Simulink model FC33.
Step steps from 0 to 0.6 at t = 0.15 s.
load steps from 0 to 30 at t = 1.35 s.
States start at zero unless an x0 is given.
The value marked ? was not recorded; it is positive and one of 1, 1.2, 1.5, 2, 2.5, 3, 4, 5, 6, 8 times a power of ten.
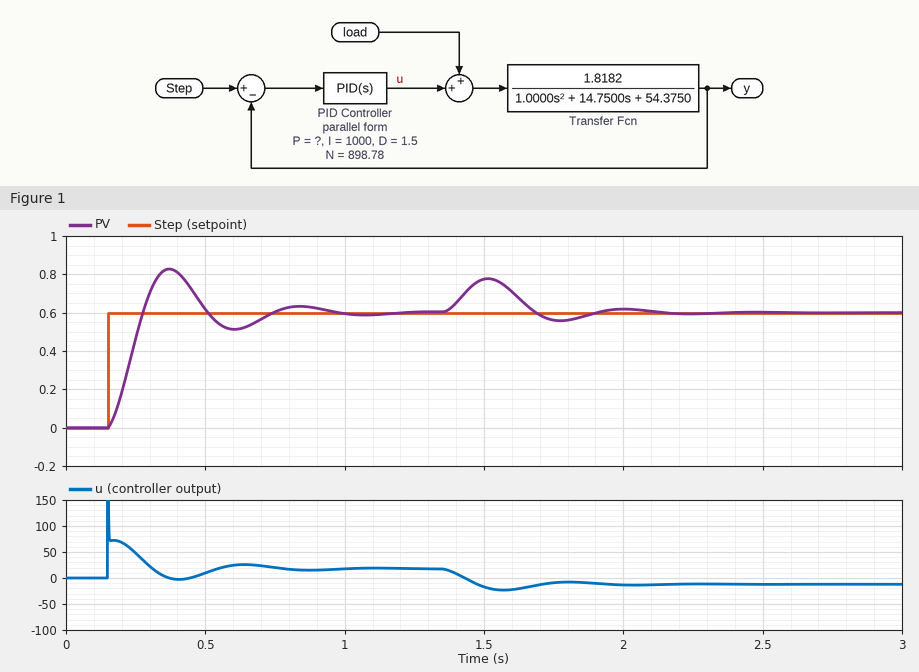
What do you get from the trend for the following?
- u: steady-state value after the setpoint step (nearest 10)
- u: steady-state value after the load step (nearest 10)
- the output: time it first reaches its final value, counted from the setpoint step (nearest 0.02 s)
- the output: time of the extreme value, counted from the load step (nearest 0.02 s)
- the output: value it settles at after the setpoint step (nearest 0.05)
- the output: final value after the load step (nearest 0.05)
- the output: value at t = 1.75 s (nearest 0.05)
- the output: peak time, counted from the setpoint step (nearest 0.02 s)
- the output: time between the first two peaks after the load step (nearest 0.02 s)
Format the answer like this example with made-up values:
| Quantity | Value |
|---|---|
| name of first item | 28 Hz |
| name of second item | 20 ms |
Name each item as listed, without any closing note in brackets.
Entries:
| Quantity | Value |
|---|---|
| u: steady-state value after the setpoint step | 20 |
| u: steady-state value after the load step | -10 |
| the output: time it first reaches its final value, counted from the setpoint step | 0.12 s |
| the output: time of the extreme value, counted from the load step | 0.16 s |
| the output: value it settles at after the setpoint step | 0.60 |
| the output: final value after the load step | 0.60 |
| the output: value at t = 1.75 s | 0.55 |
| the output: peak time, counted from the setpoint step | 0.22 s |
| the output: time between the first two peaks after the load step | 0.48 s |
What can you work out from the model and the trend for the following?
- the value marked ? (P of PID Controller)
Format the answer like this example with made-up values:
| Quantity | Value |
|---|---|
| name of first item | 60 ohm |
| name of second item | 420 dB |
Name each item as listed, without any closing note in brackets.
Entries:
| Quantity | Value |
|---|---|
| the value marked ? | 120 |
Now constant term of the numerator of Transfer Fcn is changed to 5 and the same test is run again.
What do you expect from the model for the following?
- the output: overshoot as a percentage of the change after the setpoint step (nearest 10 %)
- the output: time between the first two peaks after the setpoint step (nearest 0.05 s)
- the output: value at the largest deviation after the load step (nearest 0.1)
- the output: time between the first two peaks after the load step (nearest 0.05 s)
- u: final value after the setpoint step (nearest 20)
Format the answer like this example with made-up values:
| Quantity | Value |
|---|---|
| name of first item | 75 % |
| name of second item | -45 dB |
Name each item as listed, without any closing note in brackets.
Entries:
| Quantity | Value |
|---|---|
| the output: overshoot as a percentage of the change after the setpoint step | 40 % |
| the output: time between the first two peaks after the setpoint step | 0.30 s |
| the output: value at the largest deviation after the load step | 0.8 |
| the output: time between the first two peaks after the load step | 0.30 s |
| u: final value after the setpoint step | 0 |
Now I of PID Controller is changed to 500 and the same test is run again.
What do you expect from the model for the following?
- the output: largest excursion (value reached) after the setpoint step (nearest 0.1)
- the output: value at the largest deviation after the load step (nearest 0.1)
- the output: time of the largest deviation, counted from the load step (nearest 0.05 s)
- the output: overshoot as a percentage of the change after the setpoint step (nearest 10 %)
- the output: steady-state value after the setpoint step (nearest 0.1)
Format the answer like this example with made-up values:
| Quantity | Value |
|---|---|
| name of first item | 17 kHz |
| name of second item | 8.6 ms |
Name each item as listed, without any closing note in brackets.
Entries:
| Quantity | Value |
|---|---|
| the output: largest excursion (value reached) after the setpoint step | 0.7 |
| the output: value at the largest deviation after the load step | 0.8 |
| the output: time of the largest deviation, counted from the load step | 0.20 s |
| the output: overshoot as a percentage of the change after the setpoint step | 20 % |
| the output: steady-state value after the setpoint step | 0.6 |
